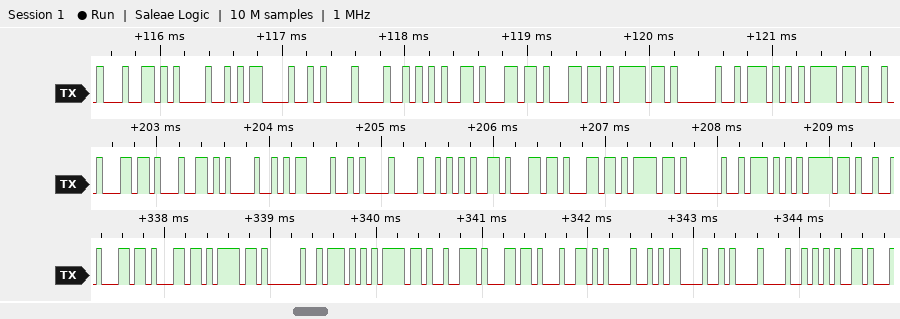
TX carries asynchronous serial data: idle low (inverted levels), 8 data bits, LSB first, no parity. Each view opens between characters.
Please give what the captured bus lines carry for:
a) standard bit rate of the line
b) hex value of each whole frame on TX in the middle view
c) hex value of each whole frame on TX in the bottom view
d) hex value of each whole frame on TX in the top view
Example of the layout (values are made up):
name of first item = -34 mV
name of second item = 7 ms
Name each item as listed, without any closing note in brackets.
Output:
standard bit rate of the line = 19200 baud
hex value of each whole frame on TX in the middle view = 27, 37, BD, E5, EB, 6F, 35, 27, 27, 21, BF, 51, 21
hex value of each whole frame on TX in the bottom view = 27, 27, 21, BF, 51, 21, 1B, 27, 37, BD, E5, EB, 6F, 35
hex value of each whole frame on TX in the top view = 37, BD, E5, EB, 6F, 35, 27, 27, 21, BF, 51, 21
